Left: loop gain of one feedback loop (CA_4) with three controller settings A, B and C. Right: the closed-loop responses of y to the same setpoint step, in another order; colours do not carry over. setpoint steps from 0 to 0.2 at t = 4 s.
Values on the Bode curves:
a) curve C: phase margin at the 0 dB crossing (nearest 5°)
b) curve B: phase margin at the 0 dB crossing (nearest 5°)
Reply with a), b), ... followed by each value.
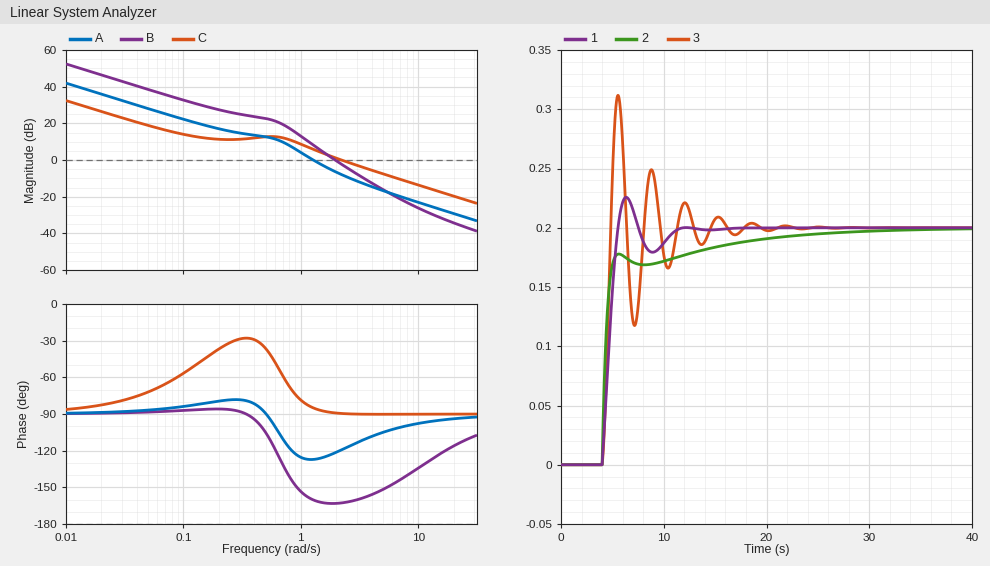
a) 90°
b) 15°
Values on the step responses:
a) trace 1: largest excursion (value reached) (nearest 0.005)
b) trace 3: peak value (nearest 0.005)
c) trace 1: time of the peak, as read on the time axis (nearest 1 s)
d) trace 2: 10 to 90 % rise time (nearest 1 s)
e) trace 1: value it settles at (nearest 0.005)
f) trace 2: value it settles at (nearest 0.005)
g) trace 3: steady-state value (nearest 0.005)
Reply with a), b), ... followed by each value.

a) 0.225
b) 0.310
c) 6 s
d) 9 s
e) 0.200
f) 0.200
g) 0.200
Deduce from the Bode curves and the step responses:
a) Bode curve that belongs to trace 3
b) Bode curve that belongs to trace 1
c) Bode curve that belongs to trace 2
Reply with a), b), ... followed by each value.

a) B
b) A
c) C
